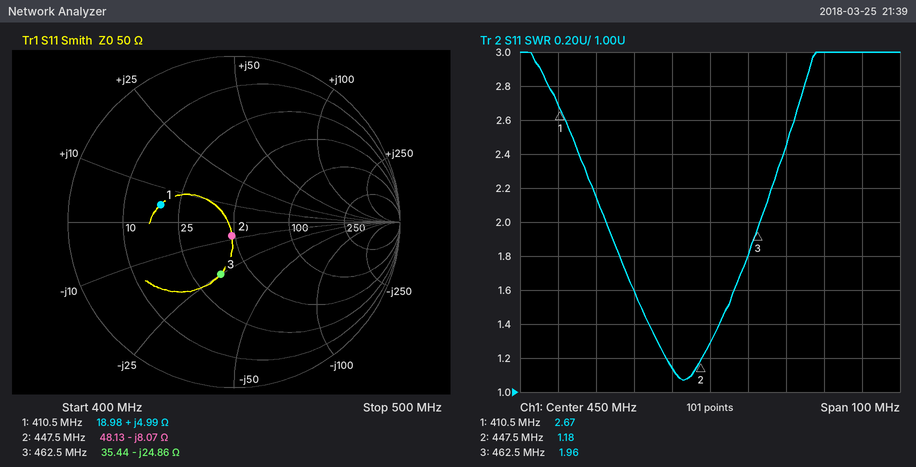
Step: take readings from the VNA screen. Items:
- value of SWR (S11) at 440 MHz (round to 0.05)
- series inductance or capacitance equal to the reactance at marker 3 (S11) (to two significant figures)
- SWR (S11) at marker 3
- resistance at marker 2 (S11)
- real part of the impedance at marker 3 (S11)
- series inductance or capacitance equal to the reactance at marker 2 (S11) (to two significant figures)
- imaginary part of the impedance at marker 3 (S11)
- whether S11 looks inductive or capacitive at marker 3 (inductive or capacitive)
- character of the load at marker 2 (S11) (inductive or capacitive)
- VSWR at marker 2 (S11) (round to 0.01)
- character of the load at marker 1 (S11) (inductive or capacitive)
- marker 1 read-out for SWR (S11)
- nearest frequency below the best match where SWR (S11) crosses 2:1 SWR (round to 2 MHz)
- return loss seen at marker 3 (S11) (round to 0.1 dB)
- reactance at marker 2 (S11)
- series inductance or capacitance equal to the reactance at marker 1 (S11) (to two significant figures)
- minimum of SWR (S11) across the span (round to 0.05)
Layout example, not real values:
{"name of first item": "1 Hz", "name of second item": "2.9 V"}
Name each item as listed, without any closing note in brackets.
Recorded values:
{"value of SWR (S11) at 440 MHz": "1.15", "series inductance or capacitance equal to the reactance at marker 3 (S11)": "14 pF", "SWR (S11) at marker 3": "1.96", "resistance at marker 2": "48.13 Ω", "real part of the impedance at marker 3": "35.44 Ω", "series inductance or capacitance equal to the reactance at marker 2 (S11)": "44 pF", "imaginary part of the impedance at marker 3": "-24.86 Ω", "whether S11 looks inductive or capacitive at marker 3": "capacitive", "character of the load at marker 2 (S11)": "capacitive", "VSWR at marker 2 (S11)": "1.18", "character of the load at marker 1 (S11)": "inductive", "marker 1 read-out for SWR": "2.67", "nearest frequency below the best match where SWR (S11) crosses 2:1 SWR": "422 MHz", "return loss seen at marker 3 (S11)": "9.8 dB", "reactance at marker 2": "-8.07 Ω", "series inductance or capacitance equal to the reactance at marker 1 (S11)": "1.9 nH", "minimum of SWR (S11) across the span": "1.05"}
